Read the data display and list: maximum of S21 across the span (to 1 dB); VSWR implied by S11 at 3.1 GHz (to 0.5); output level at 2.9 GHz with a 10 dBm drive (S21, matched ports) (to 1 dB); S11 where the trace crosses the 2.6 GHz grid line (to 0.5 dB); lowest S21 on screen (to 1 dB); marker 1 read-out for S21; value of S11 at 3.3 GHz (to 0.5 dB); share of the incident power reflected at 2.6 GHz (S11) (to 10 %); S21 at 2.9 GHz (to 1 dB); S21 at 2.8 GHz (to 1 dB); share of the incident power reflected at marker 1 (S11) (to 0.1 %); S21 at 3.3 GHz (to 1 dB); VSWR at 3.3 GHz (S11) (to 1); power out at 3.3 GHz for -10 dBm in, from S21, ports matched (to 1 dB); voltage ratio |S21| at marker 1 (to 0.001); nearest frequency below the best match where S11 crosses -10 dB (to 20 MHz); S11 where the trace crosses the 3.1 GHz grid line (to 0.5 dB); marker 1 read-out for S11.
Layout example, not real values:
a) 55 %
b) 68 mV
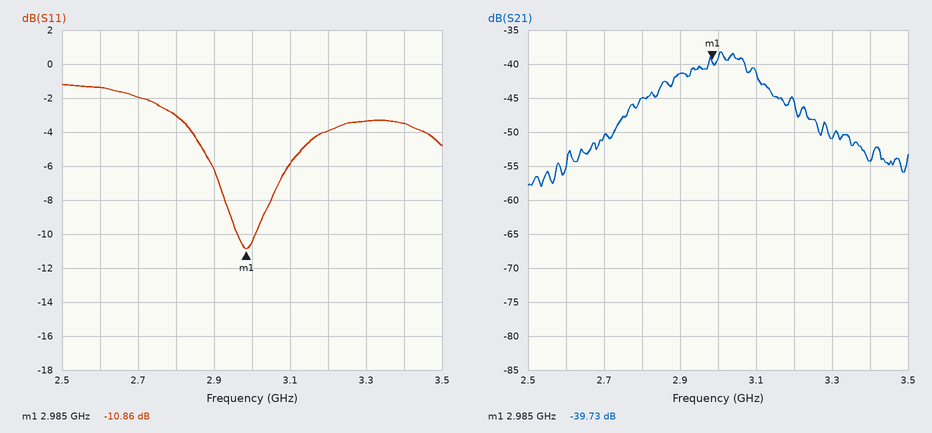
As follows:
a) -38 dB
b) 3.0
c) -31 dBm
d) -1.5 dB
e) -58 dB
f) -39.73 dB
g) -3.5 dB
h) 70 %
i) -41 dB
j) -45 dB
k) 8.2 %
l) -51 dB
m) 5
n) -61 dBm
o) 0.010
p) 2.96 GHz
q) -6.0 dB
r) -10.86 dB
